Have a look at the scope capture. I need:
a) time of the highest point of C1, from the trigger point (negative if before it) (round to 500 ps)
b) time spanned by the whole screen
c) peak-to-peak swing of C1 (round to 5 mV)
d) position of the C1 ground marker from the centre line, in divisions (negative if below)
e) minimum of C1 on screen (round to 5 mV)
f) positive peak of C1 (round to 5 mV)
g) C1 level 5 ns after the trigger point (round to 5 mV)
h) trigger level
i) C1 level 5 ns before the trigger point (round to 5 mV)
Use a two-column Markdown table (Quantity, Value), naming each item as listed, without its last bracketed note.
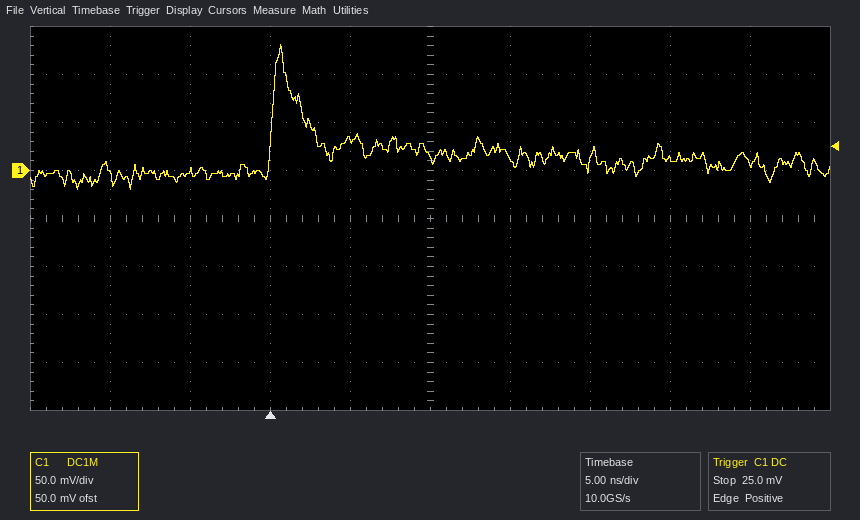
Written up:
| Quantity | Value |
|---|---|
| time of the highest point of C1, from the trigger point (negative if before it) | +500 ps |
| time spanned by the whole screen | 50 ns |
| peak-to-peak swing of C1 | 150 mV |
| position of the C1 ground marker from the centre line, in divisions | +1.0 div |
| minimum of C1 on screen | -20 mV |
| positive peak of C1 | 130 mV |
| C1 level 5 ns after the trigger point | 30 mV |
| trigger level | 25.0 mV |
| C1 level 5 ns before the trigger point | 0 mV |
